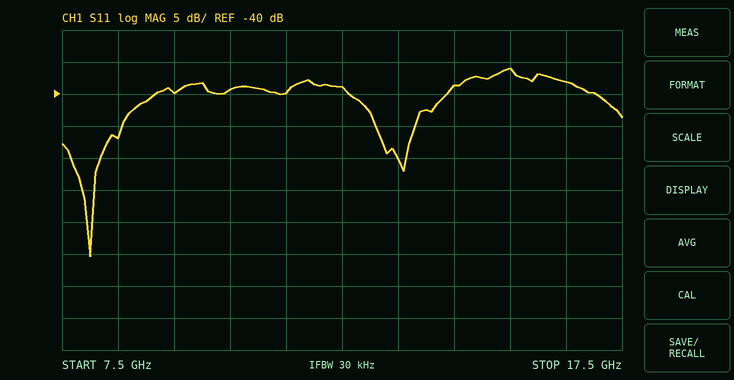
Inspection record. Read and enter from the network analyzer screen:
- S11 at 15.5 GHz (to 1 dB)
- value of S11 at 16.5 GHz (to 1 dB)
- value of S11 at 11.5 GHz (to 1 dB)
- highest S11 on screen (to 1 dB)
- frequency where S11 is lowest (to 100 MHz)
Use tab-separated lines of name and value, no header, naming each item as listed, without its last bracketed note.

S11 at 15.5 GHz	-36 dB
value of S11 at 16.5 GHz	-38 dB
value of S11 at 11.5 GHz	-40 dB
highest S11 on screen	-36 dB
frequency where S11 is lowest	8.0 GHz
